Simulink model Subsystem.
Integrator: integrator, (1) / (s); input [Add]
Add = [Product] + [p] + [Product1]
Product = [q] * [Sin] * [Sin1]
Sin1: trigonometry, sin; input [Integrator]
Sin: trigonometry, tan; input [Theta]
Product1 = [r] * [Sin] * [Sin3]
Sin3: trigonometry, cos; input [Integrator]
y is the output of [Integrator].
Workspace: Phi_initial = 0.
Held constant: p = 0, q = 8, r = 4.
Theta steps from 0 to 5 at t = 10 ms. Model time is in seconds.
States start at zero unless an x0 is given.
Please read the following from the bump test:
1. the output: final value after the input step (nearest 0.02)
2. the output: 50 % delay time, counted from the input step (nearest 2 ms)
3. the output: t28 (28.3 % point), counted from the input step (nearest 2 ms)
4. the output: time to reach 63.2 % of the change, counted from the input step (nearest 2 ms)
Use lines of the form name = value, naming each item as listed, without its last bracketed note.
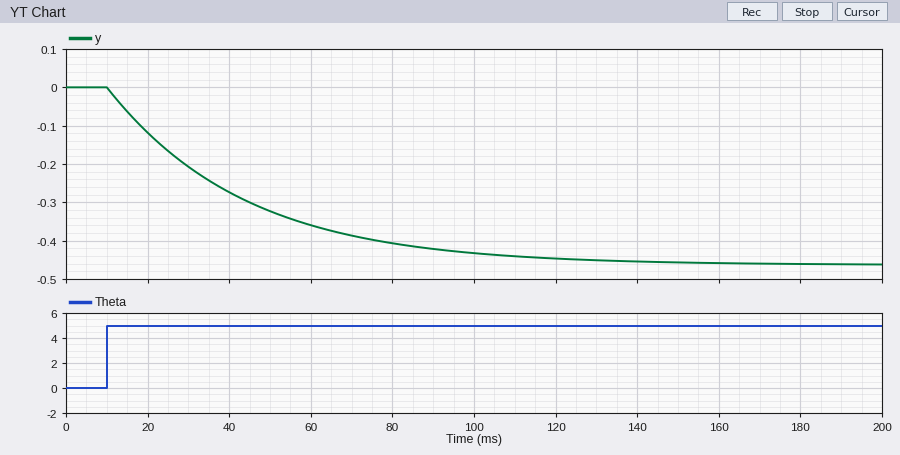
the output: final value after the input step = -0.46
the output: 50 % delay time, counted from the input step = 24 ms
the output: t28 (28.3 % point), counted from the input step = 12 ms
the output: time to reach 63.2 % of the change, counted from the input step = 34 ms
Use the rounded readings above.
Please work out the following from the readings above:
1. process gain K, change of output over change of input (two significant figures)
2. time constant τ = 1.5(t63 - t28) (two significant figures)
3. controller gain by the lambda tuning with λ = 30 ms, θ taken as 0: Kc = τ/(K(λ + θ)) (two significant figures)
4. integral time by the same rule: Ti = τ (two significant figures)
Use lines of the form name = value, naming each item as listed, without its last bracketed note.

process gain K, change of output over change of input = -0.092
time constant τ = 1.5(t63 - t28) = 33 ms
controller gain by the lambda tuning with λ = 30 ms, θ taken as 0: Kc = τ/(K(λ + θ)) = -12
integral time by the same rule: Ti = τ = 33 ms
